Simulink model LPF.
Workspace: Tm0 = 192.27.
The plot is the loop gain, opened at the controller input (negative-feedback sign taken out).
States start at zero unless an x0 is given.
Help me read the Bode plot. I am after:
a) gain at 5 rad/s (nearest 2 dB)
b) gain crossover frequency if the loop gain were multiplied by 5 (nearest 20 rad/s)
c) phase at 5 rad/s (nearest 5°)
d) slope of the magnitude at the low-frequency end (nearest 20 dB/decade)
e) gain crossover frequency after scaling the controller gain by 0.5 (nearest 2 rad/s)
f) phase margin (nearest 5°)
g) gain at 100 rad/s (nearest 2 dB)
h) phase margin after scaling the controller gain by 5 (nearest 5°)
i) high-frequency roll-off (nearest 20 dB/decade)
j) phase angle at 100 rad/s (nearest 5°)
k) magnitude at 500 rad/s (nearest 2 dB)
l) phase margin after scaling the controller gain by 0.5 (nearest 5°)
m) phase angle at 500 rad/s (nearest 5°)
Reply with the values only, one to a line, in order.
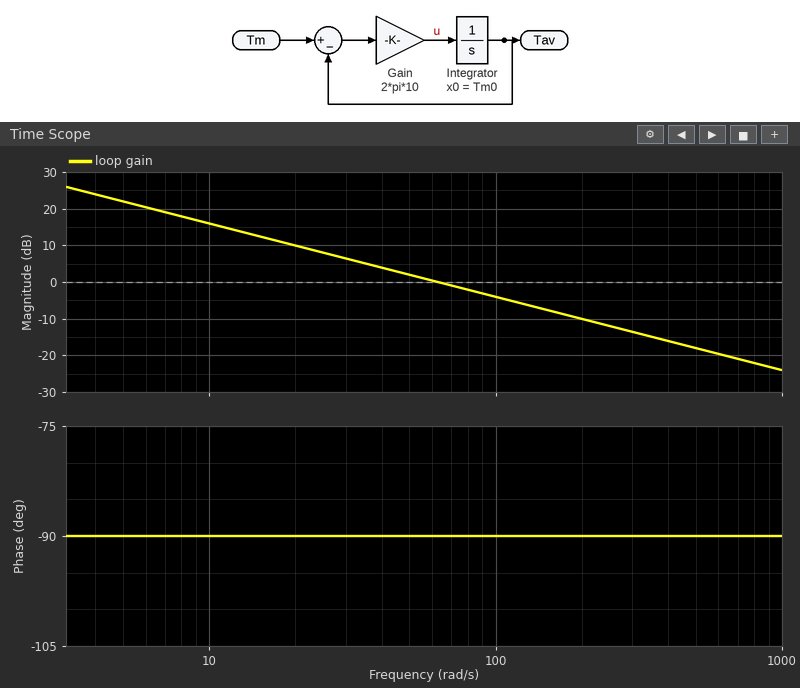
22 dB
320 rad/s
-90°
-20 dB/decade
32 rad/s
90°
-4 dB
90°
-20 dB/decade
-90°
-18 dB
90°
-90°
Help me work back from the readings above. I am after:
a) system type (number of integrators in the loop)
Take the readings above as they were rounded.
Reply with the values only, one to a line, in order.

1
